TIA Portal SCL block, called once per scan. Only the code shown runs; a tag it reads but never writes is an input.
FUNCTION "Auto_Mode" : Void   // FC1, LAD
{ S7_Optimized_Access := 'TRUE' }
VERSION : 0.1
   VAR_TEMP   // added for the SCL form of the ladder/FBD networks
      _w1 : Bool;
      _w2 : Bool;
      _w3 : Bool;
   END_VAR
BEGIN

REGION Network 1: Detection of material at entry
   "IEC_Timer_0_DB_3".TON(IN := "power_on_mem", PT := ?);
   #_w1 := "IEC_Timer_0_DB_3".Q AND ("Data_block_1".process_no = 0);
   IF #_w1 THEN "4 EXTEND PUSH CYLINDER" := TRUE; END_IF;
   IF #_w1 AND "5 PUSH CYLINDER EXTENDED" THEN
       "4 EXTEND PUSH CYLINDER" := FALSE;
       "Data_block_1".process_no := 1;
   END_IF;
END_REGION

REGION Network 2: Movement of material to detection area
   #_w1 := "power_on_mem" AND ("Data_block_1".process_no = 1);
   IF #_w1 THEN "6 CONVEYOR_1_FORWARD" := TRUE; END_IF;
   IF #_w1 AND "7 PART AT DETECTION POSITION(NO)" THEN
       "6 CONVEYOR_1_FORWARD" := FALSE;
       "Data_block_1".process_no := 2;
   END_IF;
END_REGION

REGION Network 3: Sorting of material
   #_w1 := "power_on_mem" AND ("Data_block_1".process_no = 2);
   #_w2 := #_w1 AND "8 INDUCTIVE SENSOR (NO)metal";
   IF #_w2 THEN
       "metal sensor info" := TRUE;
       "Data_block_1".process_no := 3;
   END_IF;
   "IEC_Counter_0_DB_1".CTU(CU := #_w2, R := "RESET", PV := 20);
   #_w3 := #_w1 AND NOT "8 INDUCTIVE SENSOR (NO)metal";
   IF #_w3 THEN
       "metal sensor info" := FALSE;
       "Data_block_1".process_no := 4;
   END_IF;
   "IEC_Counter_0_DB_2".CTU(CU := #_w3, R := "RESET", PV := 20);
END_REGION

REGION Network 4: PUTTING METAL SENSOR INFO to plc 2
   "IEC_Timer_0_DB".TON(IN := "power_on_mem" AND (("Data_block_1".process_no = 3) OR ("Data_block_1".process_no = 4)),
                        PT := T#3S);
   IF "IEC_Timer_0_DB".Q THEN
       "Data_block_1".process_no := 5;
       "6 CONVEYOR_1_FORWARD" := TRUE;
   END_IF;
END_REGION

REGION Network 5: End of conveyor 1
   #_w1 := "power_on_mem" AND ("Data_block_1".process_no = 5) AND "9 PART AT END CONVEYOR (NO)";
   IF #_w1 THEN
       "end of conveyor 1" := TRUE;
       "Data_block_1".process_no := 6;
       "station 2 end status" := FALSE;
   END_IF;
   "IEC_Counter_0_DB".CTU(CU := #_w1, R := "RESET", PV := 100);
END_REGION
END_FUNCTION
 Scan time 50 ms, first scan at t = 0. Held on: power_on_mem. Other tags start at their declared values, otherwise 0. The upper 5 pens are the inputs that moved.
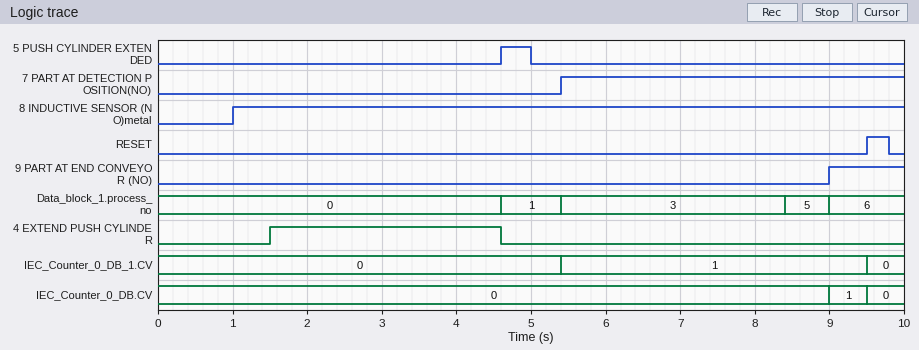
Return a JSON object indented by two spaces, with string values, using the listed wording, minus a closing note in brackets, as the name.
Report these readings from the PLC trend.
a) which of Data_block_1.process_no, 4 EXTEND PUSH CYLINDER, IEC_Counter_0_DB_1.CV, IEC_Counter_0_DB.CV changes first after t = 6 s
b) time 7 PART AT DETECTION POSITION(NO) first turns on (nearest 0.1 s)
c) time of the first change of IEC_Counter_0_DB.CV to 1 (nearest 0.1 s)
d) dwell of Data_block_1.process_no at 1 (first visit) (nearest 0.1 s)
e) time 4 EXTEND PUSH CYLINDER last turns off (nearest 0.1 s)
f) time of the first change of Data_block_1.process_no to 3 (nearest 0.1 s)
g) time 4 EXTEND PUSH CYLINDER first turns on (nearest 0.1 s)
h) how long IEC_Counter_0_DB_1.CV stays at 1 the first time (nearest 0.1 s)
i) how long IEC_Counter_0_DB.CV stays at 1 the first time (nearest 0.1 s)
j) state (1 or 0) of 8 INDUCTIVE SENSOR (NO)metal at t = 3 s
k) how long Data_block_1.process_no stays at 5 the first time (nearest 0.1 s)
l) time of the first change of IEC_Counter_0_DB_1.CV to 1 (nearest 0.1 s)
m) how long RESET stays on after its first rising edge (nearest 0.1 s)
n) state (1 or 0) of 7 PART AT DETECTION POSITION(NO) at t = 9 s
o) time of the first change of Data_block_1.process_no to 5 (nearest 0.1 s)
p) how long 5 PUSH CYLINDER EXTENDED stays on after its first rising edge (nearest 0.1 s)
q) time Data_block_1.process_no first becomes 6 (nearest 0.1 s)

{
  "which of Data_block_1.process_no, 4 EXTEND PUSH CYLINDER, IEC_Counter_0_DB_1.CV, IEC_Counter_0_DB.CV changes first after t = 6 s": "Data_block_1.process_no",
  "time 7 PART AT DETECTION POSITION(NO) first turns on": "5.4 s",
  "time of the first change of IEC_Counter_0_DB.CV to 1": "9.0 s",
  "dwell of Data_block_1.process_no at 1 (first visit)": "0.8 s",
  "time 4 EXTEND PUSH CYLINDER last turns off": "4.6 s",
  "time of the first change of Data_block_1.process_no to 3": "5.4 s",
  "time 4 EXTEND PUSH CYLINDER first turns on": "1.5 s",
  "how long IEC_Counter_0_DB_1.CV stays at 1 the first time": "4.1 s",
  "how long IEC_Counter_0_DB.CV stays at 1 the first time": "0.5 s",
  "state (1 or 0) of 8 INDUCTIVE SENSOR (NO)metal at t = 3 s": "1",
  "how long Data_block_1.process_no stays at 5 the first time": "0.6 s",
  "time of the first change of IEC_Counter_0_DB_1.CV to 1": "5.4 s",
  "how long RESET stays on after its first rising edge": "0.3 s",
  "state (1 or 0) of 7 PART AT DETECTION POSITION(NO) at t = 9 s": "1",
  "time of the first change of Data_block_1.process_no to 5": "8.4 s",
  "how long 5 PUSH CYLINDER EXTENDED stays on after its first rising edge": "0.4 s",
  "time Data_block_1.process_no first becomes 6": "9.0 s"
}
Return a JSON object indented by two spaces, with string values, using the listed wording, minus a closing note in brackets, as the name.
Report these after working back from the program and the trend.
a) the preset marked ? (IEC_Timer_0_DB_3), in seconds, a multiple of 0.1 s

{
  "the preset marked ? (IEC_Timer_0_DB_3), in seconds, a multiple of 0.1 s": "1.5 s"
}
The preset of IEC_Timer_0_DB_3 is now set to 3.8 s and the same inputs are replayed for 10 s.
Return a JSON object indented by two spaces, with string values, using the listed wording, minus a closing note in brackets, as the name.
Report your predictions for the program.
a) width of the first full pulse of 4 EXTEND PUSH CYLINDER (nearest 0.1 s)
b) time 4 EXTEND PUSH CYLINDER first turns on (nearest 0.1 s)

{
  "width of the first full pulse of 4 EXTEND PUSH CYLINDER": "0.8 s",
  "time 4 EXTEND PUSH CYLINDER first turns on": "3.8 s"
}
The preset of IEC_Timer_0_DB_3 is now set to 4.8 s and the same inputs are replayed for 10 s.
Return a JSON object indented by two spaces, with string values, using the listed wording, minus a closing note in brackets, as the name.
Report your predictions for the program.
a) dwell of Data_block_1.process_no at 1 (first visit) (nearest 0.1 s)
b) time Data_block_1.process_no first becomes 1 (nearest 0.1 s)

{
  "dwell of Data_block_1.process_no at 1 (first visit)": "0.6 s",
  "time Data_block_1.process_no first becomes 1": "4.8 s"
}
